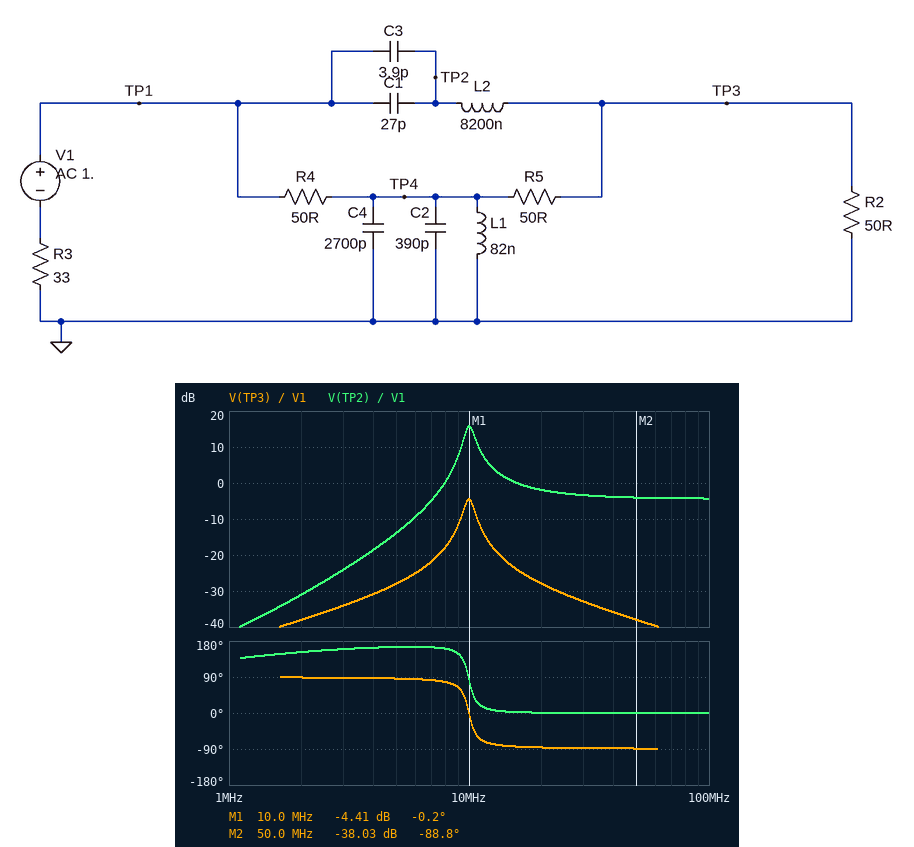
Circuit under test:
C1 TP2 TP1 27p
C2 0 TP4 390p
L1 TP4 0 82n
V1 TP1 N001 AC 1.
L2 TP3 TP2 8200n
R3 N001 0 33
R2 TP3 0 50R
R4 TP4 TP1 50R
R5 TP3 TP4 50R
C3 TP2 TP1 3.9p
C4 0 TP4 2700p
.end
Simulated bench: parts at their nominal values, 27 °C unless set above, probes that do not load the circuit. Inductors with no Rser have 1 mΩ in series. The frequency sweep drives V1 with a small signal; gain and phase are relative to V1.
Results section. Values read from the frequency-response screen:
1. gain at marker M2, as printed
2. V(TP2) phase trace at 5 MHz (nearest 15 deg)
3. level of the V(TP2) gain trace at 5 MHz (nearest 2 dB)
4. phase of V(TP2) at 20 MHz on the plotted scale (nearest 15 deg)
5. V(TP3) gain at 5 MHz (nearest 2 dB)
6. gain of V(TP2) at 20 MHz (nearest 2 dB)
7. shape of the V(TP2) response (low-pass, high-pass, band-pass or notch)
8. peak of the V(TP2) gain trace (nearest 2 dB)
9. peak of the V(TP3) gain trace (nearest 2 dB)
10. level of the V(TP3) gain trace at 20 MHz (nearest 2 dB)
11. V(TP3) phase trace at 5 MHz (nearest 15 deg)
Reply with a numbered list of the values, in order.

1. -38.03 dB
2. 165 deg
3. -14 dB
4. 0 deg
5. -28 dB
6. -2 dB
7. high-pass
8. 16 dB
9. -4 dB
10. -28 dB
11. 90 deg
